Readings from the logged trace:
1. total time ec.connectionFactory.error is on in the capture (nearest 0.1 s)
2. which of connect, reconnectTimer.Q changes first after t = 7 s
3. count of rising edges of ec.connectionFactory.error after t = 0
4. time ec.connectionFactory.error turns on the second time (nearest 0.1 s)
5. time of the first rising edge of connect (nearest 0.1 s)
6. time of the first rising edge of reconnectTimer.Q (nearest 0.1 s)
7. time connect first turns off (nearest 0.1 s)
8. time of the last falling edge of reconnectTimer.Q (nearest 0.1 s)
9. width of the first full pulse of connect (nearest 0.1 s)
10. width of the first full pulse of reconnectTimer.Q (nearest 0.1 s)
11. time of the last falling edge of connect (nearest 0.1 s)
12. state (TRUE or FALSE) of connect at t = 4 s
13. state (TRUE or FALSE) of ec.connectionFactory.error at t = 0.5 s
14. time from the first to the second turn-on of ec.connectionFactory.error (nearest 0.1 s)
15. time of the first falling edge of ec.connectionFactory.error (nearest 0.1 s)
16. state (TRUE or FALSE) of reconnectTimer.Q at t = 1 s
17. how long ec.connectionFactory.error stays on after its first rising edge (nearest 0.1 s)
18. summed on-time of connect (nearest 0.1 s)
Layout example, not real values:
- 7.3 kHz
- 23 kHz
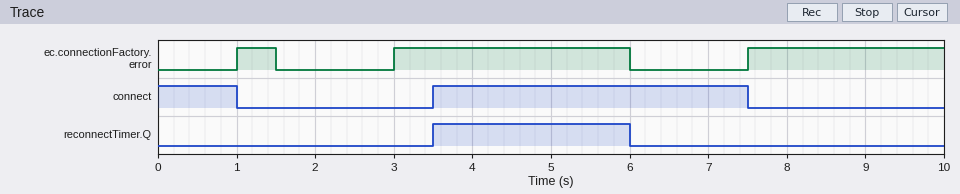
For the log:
- 6.0 s
- connect
- 3
- 3.0 s
- 3.5 s
- 3.5 s
- 1.0 s
- 6.0 s
- 4.0 s
- 2.5 s
- 7.5 s
- TRUE
- FALSE
- 2.0 s
- 1.5 s
- FALSE
- 0.5 s
- 5.0 s
